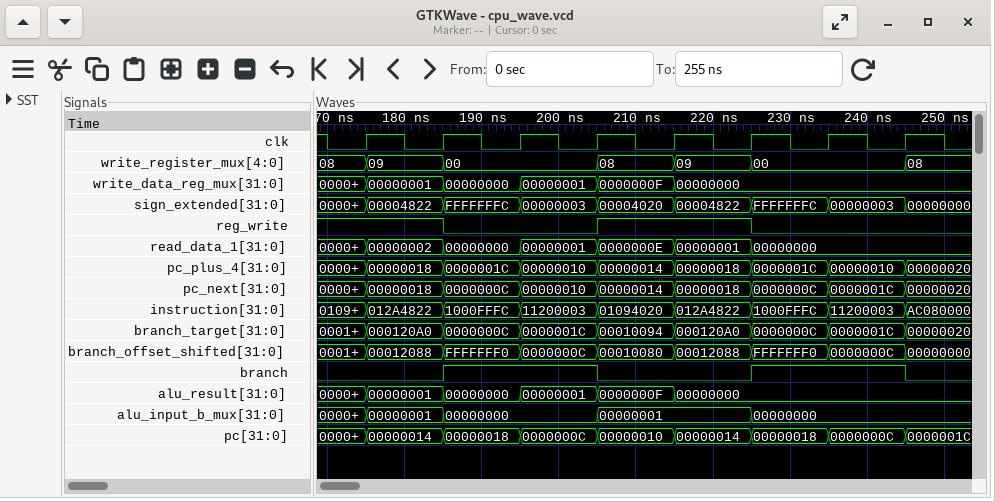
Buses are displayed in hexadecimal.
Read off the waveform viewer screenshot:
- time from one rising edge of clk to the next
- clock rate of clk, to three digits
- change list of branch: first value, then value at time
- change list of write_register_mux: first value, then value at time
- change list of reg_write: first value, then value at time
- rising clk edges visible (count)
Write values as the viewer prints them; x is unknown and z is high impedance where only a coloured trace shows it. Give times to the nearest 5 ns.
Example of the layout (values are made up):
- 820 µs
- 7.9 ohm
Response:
- 10 ns
- 100 MHz
- 0, 1 at 185 ns, 0 at 205 ns, 1 at 225 ns, 0 at 245 ns
- 08, 09 at 175 ns, 00 at 185 ns, 08 at 205 ns, 09 at 215 ns, 00 at 225 ns, 08 at 245 ns
- 1, 0 at 185 ns, 1 at 205 ns, 0 at 225 ns
- 8
